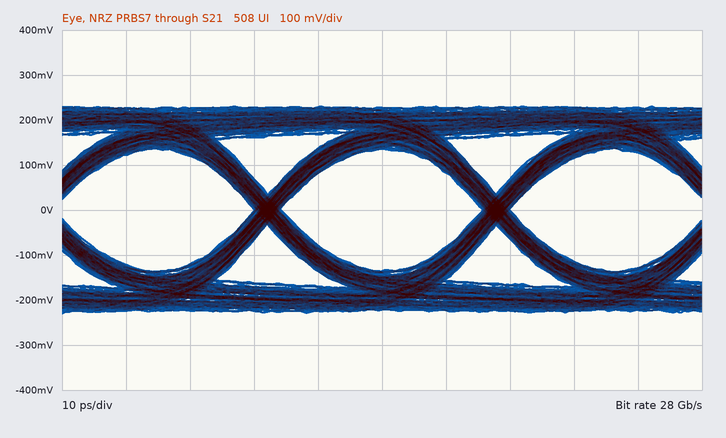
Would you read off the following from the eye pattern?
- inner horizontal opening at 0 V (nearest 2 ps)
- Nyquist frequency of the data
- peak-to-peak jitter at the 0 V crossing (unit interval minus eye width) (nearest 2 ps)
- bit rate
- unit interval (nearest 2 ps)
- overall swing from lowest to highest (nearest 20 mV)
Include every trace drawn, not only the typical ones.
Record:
32 ps
14 GHz
4 ps
28 Gb/s
36 ps
460 mV
